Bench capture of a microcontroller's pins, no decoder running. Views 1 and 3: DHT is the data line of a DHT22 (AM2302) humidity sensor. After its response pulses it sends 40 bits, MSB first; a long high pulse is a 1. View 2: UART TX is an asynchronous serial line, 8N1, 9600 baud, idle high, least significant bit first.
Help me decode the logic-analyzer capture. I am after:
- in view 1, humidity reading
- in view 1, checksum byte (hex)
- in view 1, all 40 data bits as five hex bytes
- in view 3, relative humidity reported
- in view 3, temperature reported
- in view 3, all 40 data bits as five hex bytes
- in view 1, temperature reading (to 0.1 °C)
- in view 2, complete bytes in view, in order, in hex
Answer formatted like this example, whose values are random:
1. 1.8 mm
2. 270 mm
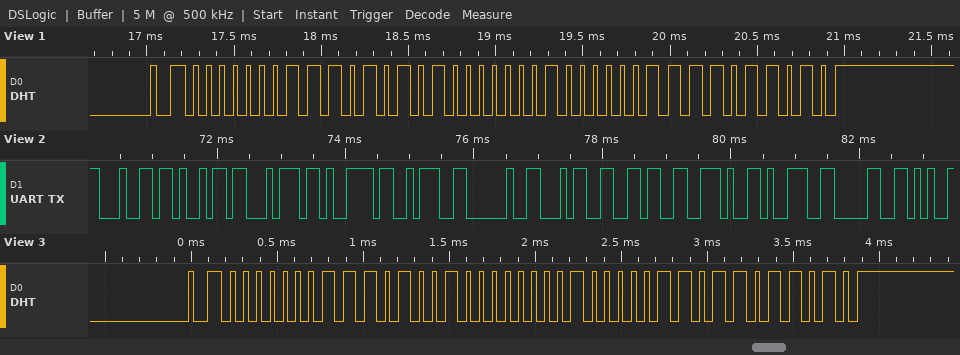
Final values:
1. 46.9 %
2. 0xDA
3. 01 D5 01 03 DA
4. 46.6 %
5. 26.2 °C
6. 01 D2 01 06 DA
7. 25.9 °C
8. 64 69 74 79 3A 20 34 36 2E 39 30
